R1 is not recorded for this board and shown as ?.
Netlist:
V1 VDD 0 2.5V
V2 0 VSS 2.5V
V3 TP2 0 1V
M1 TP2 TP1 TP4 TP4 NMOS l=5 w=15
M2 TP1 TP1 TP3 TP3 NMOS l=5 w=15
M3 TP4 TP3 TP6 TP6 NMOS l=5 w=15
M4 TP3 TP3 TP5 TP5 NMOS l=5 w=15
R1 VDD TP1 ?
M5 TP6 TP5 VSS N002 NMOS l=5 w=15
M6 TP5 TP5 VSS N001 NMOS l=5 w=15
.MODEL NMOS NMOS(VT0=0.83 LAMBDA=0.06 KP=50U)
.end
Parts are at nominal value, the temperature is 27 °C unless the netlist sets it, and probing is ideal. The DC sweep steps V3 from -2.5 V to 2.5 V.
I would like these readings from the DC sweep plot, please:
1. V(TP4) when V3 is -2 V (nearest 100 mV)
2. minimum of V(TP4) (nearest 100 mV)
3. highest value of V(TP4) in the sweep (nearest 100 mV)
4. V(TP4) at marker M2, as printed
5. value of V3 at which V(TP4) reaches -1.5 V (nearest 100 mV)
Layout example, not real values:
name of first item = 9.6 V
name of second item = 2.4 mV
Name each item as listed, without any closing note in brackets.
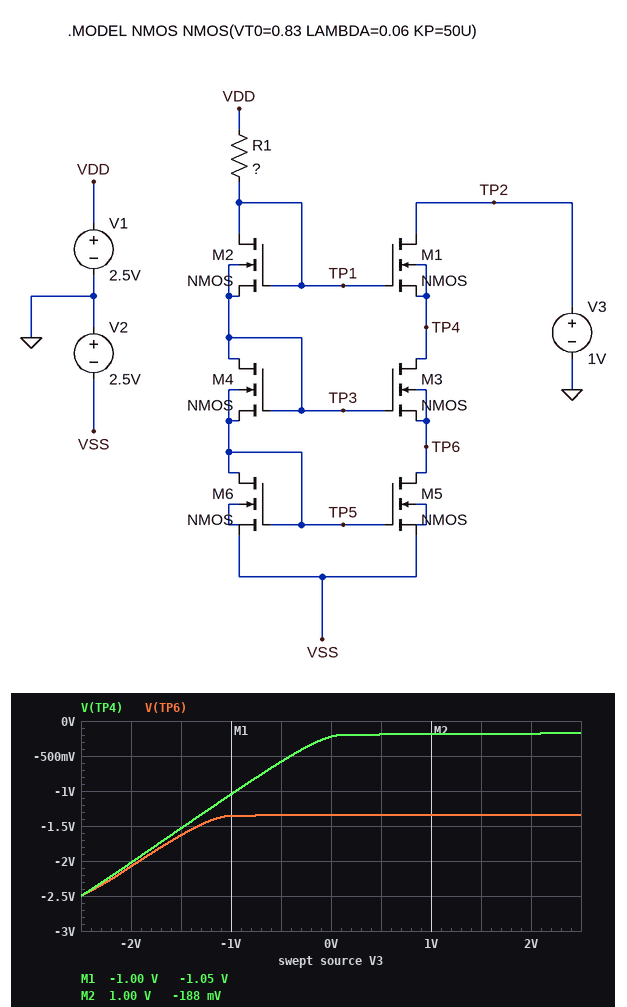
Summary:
V(TP4) when V3 is -2 V = -2.0 V
minimum of V(TP4) = -2.5 V
highest value of V(TP4) in the sweep = -200 mV
V(TP4) at marker M2, as printed = -188 mV
value of V3 at which V(TP4) reaches -1.5 V = -1.5 V
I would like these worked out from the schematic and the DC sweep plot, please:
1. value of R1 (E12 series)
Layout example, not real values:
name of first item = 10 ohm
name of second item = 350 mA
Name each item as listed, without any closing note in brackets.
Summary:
value of R1 = 180 kΩ
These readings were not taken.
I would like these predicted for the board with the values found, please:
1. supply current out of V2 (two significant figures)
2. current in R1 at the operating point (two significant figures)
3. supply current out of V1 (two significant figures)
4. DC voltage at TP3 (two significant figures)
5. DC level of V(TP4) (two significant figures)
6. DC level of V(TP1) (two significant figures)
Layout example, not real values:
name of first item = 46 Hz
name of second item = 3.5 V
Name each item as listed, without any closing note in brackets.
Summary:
supply current out of V2 = 17 µA
current in R1 at the operating point = 8.5 µA
supply current out of V1 = 8.5 µA
DC voltage at TP3 = -190 mV
DC level of V(TP4) = -190 mV
DC level of V(TP1) = 970 mV
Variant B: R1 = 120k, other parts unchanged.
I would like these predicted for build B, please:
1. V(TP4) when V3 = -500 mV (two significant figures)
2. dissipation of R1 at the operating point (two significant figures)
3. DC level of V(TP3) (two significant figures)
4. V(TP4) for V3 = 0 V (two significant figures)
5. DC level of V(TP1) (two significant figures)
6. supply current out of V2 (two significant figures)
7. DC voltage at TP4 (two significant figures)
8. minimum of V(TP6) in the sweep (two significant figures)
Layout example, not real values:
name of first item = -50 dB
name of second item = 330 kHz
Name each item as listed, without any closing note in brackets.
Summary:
V(TP4) when V3 = -500 mV = -590 mV
dissipation of R1 at the operating point = 16 µW
DC level of V(TP3) = -85 mV
V(TP4) for V3 = 0 V = -190 mV
DC level of V(TP1) = 1.1 V
supply current out of V2 = 23 µA
DC voltage at TP4 = -86 mV
minimum of V(TP6) in the sweep = -2.5 V
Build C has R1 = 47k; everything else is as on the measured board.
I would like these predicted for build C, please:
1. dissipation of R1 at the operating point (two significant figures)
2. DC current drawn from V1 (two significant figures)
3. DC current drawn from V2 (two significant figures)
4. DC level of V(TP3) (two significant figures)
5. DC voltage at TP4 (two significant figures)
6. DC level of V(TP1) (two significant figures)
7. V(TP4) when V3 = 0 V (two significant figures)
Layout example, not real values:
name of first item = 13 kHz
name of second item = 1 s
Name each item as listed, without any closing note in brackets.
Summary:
dissipation of R1 at the operating point = 21 µW
DC current drawn from V1 = 21 µA
DC current drawn from V2 = 42 µA
DC level of V(TP3) = 180 mV
DC voltage at TP4 = 170 mV
DC level of V(TP1) = 1.5 V
V(TP4) when V3 = 0 V = -180 mV
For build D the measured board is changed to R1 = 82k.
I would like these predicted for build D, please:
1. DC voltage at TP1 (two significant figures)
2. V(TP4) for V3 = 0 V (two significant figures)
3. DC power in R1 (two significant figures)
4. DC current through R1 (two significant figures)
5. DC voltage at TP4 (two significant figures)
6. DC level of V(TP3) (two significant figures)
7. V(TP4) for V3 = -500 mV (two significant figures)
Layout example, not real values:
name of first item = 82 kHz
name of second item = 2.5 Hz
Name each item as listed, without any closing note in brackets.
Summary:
DC voltage at TP1 = 1.3 V
V(TP4) for V3 = 0 V = -180 mV
DC power in R1 = 18 µW
DC current through R1 = 15 µA
DC voltage at TP4 = 16 mV
DC level of V(TP3) = 19 mV
V(TP4) for V3 = -500 mV = -600 mV
